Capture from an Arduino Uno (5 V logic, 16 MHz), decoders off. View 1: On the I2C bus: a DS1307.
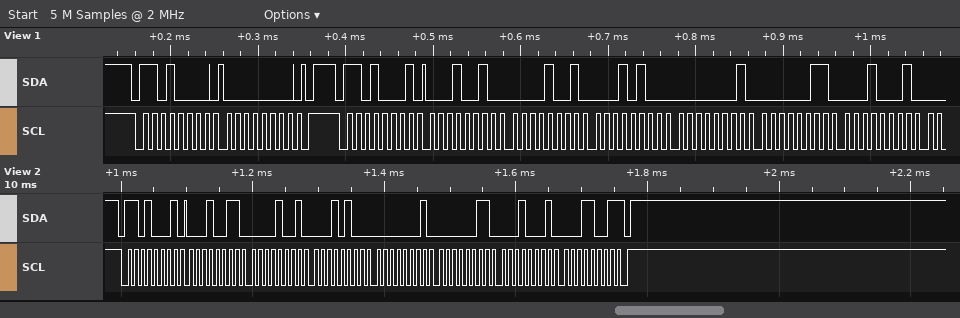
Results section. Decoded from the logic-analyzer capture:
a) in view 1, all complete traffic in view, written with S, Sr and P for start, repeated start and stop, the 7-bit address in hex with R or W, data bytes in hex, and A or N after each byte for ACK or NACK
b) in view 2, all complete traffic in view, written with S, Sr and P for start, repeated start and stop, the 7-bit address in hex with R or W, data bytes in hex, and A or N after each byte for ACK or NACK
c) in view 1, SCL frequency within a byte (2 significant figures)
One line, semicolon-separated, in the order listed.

S 68W A 00 A P S 68R A 12 A 09 A 14 A 01 A 03 A 11 A; S 68R A 13 A 09 A 14 A 01 A 03 A 11 A 19 N P; 100 kHz
